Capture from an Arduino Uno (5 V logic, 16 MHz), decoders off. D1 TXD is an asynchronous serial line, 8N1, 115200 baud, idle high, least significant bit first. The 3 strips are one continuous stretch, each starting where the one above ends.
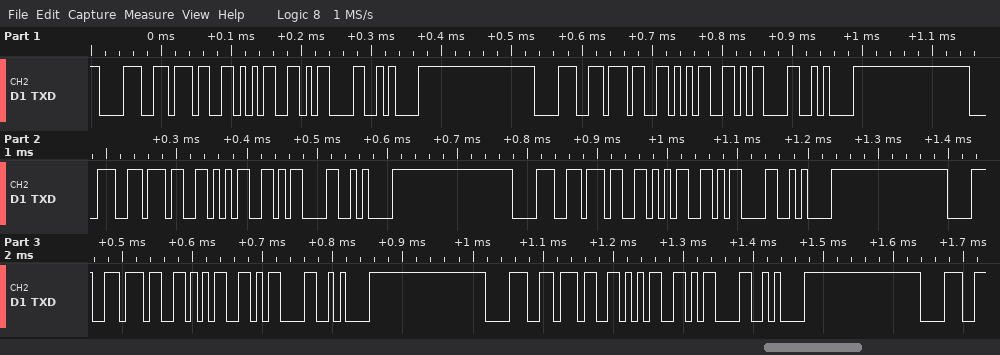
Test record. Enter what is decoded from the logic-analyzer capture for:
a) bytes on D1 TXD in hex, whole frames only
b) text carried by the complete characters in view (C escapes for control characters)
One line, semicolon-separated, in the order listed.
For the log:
38 37 35 0D 0A 38 37 35 0D 0A 38 37 35 0D 0A 38 37 35 0D 0A 38 37 35 0D 0A 38 37 35 0D 0A 38; "875\r\n875\r\n875\r\n875\r\n875\r\n875\r\n8"
